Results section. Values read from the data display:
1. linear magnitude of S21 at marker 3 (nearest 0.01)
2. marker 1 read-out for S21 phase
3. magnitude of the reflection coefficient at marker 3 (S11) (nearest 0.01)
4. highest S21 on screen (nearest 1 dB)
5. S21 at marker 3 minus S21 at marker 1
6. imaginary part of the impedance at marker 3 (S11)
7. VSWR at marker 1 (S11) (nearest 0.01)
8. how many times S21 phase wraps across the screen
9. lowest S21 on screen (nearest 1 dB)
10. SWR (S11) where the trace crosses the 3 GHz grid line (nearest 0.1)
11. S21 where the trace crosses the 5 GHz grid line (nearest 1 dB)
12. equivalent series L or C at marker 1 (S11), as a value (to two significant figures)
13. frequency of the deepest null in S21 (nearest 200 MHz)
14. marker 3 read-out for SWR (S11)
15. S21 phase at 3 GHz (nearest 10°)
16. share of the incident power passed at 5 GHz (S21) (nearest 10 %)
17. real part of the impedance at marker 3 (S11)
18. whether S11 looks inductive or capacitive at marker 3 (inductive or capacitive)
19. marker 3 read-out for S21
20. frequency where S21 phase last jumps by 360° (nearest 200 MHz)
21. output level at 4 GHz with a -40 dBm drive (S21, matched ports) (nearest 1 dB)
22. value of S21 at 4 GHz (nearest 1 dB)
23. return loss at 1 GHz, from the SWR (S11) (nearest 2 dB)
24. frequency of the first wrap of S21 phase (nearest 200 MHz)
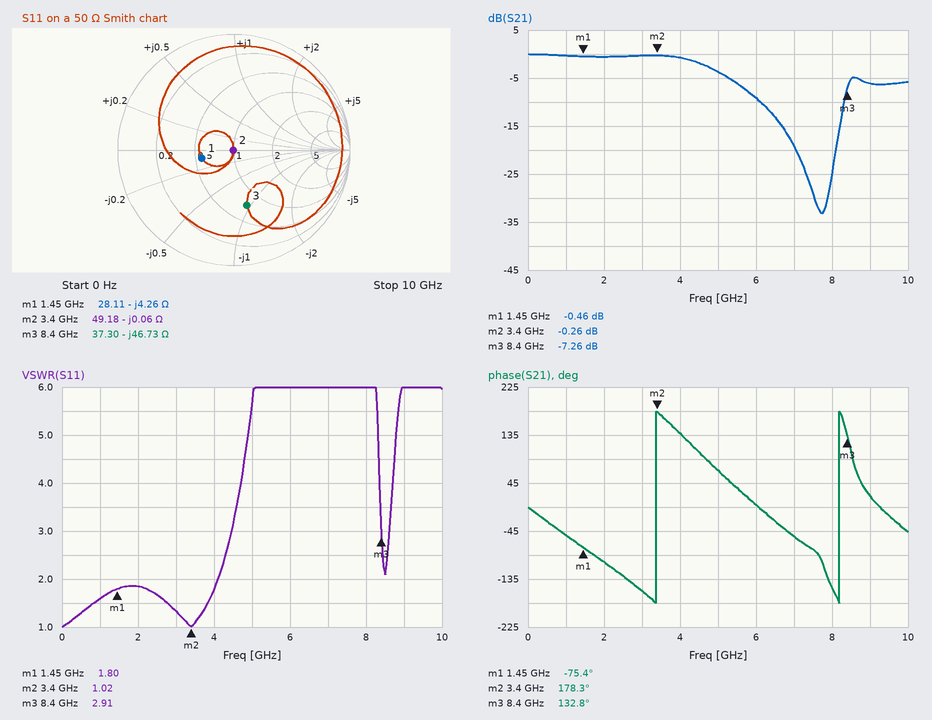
0.43
-75.4°
0.49
0 dB
-6.80 dB
-46.73 Ω
1.80
2
-33 dB
1.3
-4 dB
26 pF
7.8 GHz
2.91
-160°
40 %
37.30 Ω
capacitive
-7.26 dB
8.2 GHz
-41 dBm
-1 dB
12 dB
3.4 GHz
